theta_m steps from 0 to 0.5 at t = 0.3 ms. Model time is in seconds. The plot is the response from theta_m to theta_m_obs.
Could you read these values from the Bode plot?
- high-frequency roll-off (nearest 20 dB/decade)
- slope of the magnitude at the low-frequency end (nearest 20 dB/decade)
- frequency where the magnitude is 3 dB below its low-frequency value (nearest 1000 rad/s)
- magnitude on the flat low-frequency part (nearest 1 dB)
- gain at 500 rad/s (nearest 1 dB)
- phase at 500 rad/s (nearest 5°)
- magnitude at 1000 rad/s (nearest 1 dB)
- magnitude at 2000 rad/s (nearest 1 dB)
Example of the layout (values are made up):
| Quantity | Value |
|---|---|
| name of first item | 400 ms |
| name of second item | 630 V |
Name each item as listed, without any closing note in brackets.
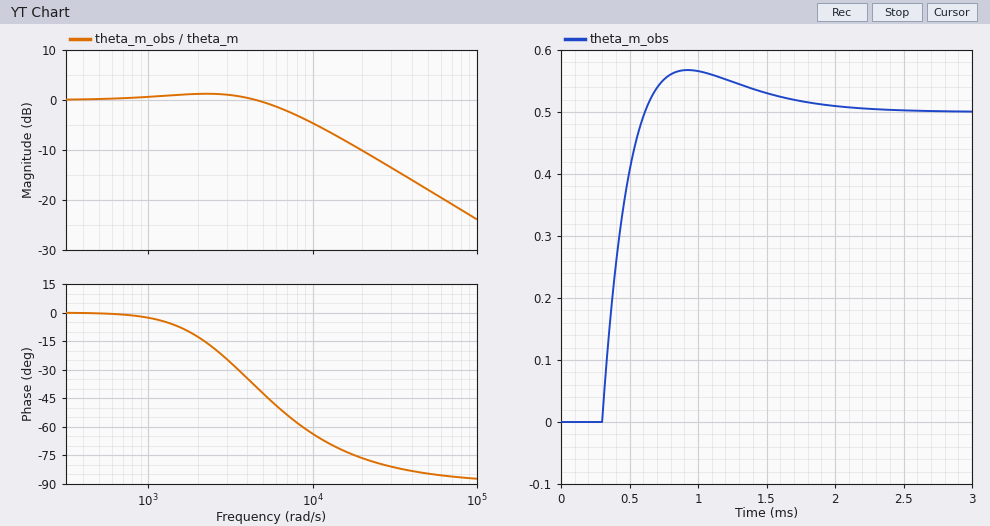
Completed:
| Quantity | Value |
|---|---|
| high-frequency roll-off | -20 dB/decade |
| slope of the magnitude at the low-frequency end | 0 dB/decade |
| frequency where the magnitude is 3 dB below its low-frequency value | 8000 rad/s |
| magnitude on the flat low-frequency part | 0 dB |
| gain at 500 rad/s | 0 dB |
| phase at 500 rad/s | 0° |
| magnitude at 1000 rad/s | 1 dB |
| magnitude at 2000 rad/s | 1 dB |
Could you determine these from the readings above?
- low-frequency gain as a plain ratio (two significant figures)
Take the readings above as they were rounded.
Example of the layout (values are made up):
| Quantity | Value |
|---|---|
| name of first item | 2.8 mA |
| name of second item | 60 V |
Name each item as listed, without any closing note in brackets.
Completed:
| Quantity | Value |
|---|---|
| low-frequency gain as a plain ratio | 1.0 |
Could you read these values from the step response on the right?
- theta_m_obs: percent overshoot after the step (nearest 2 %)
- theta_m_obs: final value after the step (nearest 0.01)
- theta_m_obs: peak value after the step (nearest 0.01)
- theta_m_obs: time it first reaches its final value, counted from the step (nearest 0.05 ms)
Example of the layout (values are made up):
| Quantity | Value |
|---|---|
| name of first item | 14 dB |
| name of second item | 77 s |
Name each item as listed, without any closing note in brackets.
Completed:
| Quantity | Value |
|---|---|
| theta_m_obs: percent overshoot after the step | 14 % |
| theta_m_obs: final value after the step | 0.50 |
| theta_m_obs: peak value after the step | 0.57 |
| theta_m_obs: time it first reaches its final value, counted from the step | 0.30 ms |
